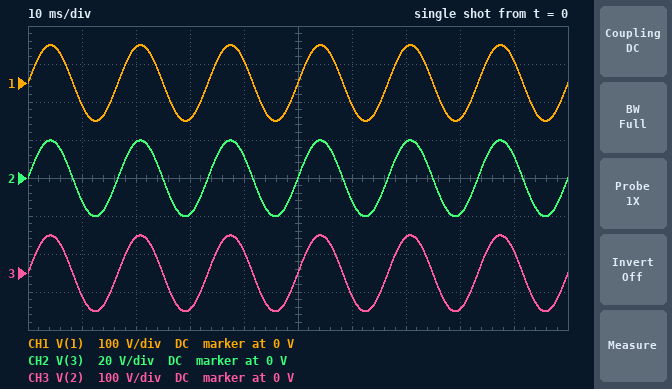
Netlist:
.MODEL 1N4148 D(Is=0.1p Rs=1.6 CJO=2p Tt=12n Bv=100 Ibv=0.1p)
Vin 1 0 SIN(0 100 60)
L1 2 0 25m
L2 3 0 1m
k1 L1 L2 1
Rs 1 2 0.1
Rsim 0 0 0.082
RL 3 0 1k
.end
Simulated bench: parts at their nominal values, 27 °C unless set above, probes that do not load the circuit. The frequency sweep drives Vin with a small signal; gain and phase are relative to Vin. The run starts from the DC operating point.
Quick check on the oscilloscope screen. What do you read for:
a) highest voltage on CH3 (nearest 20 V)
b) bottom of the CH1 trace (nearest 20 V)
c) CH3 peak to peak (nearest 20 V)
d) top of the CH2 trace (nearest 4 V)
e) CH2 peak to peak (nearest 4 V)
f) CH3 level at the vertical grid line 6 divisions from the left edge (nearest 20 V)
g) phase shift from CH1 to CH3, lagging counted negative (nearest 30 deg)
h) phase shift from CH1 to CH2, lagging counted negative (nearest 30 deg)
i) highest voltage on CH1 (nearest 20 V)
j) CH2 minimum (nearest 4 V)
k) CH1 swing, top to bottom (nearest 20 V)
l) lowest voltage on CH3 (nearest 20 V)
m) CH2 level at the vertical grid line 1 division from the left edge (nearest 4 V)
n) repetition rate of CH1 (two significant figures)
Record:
100 V
-100 V
200 V
20 V
40 V
-60 V
0 deg
0 deg
100 V
-20 V
200 V
-100 V
-12 V
60 Hz
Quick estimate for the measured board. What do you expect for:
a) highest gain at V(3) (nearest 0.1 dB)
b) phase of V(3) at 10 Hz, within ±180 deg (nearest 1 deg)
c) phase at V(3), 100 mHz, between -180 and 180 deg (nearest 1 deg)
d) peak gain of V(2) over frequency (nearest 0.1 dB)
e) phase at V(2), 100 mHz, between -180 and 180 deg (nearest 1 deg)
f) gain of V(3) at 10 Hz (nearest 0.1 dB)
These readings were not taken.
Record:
-14.0 dB
4 deg
81 deg
0 dB
81 deg
-14.0 dB
